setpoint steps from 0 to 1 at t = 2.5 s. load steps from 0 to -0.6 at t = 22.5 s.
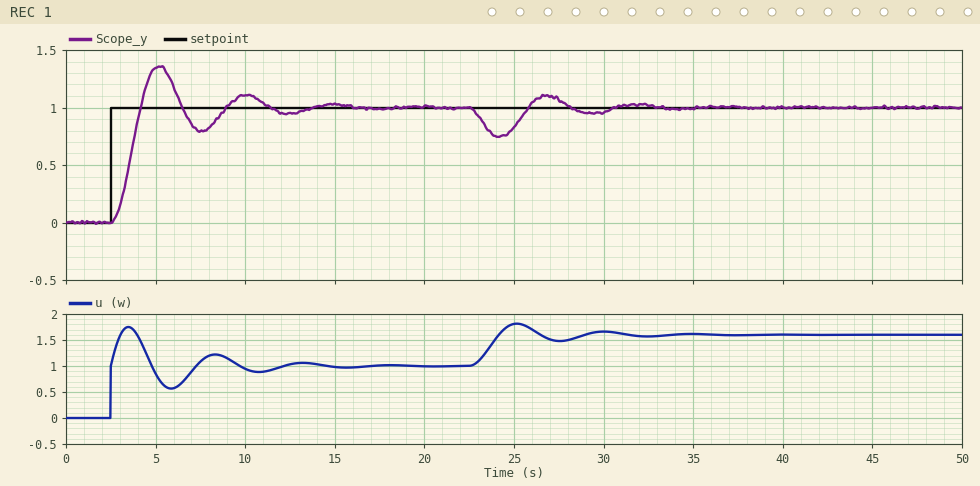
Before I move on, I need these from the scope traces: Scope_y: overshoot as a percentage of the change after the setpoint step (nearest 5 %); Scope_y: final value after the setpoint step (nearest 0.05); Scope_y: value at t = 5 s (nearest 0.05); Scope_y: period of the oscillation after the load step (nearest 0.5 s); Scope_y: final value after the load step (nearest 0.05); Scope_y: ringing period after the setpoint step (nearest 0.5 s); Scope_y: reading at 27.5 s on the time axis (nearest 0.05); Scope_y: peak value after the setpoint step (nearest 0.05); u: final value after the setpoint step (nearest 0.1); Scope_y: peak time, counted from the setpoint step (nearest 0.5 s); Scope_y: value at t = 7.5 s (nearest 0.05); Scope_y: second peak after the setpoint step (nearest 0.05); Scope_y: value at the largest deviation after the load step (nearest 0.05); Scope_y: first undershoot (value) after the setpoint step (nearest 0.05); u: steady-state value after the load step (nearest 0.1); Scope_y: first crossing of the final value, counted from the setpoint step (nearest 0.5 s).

35 %
1.00
1.35
5.0 s
1.00
5.0 s
1.05
1.35
1.0
2.5 s
0.80
1.10
0.75
0.80
1.6
1.5 s
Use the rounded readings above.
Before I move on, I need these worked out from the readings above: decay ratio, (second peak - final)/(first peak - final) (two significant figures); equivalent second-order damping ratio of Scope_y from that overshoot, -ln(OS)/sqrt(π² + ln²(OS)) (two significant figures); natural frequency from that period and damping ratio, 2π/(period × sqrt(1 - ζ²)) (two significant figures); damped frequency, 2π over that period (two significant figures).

0.29
0.32
1.3 rad/s
1.3 rad/s
